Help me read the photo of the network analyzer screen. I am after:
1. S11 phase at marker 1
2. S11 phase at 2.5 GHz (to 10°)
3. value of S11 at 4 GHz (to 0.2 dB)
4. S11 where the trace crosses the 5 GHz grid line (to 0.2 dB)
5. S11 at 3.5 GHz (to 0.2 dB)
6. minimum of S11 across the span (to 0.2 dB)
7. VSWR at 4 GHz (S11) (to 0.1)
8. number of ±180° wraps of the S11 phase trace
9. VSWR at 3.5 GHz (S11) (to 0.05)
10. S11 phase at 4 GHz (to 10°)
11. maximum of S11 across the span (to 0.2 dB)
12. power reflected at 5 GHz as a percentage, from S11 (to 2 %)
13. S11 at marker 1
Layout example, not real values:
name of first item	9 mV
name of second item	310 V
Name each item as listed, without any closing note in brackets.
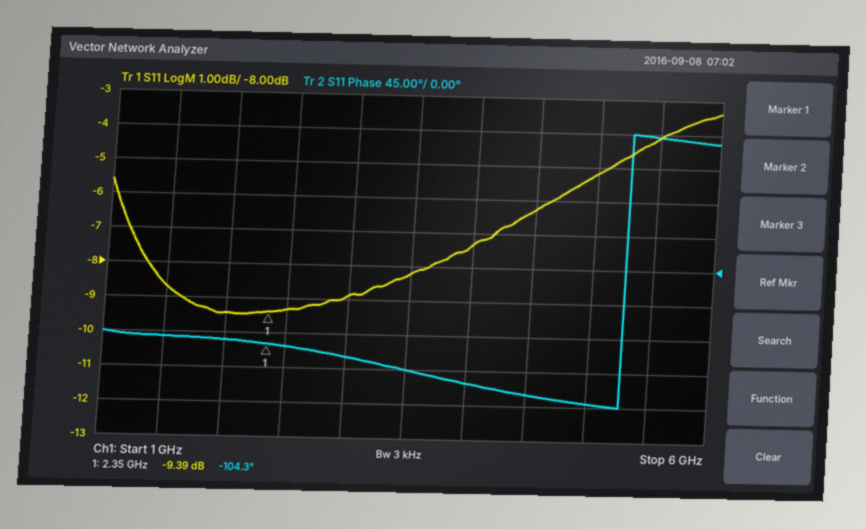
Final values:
S11 phase at marker 1	-104.3°
S11 phase at 2.5 GHz	-110°
value of S11 at 4 GHz	-7.4 dB
S11 where the trace crosses the 5 GHz grid line	-5.2 dB
S11 at 3.5 GHz	-8.2 dB
minimum of S11 across the span	-9.4 dB
VSWR at 4 GHz (S11)	2.5
number of ±180° wraps of the S11 phase trace	1
VSWR at 3.5 GHz (S11)	2.25
S11 phase at 4 GHz	-150°
maximum of S11 across the span	-3.4 dB
power reflected at 5 GHz as a percentage, from S11	30 %
S11 at marker 1	-9.39 dB
